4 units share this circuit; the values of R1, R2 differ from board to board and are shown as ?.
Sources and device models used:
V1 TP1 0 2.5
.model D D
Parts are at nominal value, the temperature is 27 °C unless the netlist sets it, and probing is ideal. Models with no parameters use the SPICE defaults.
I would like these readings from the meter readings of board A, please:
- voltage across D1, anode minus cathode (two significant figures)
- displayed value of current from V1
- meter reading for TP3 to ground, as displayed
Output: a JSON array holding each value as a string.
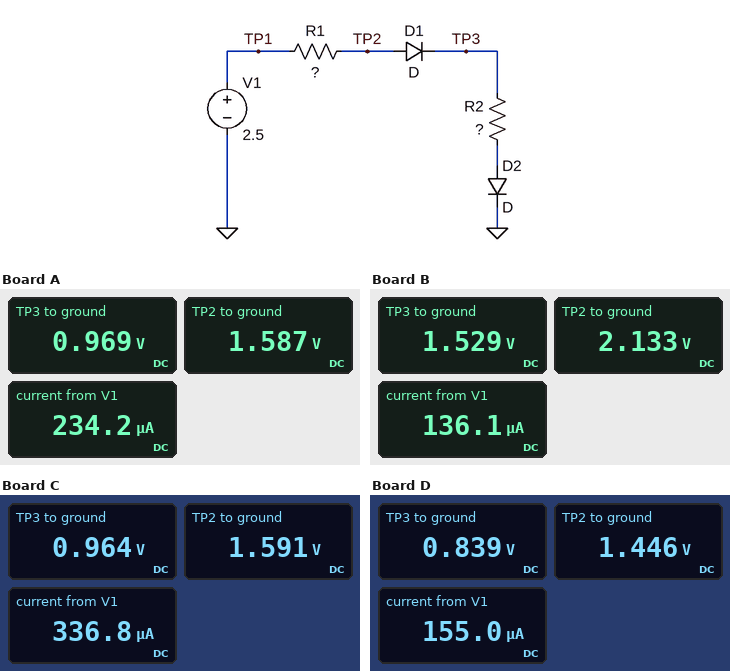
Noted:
["620 mV", "234.2 µA", "0.969 V"]
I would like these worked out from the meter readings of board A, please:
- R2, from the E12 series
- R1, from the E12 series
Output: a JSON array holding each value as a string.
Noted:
["1.5 kΩ", "3.9 kΩ"]
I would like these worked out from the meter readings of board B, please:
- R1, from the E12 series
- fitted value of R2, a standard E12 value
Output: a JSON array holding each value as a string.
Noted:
["2.7 kΩ", "6.8 kΩ"]
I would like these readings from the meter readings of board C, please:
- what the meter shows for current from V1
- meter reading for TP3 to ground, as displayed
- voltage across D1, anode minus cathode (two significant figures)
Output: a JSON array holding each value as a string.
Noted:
["336.8 µA", "0.964 V", "630 mV"]
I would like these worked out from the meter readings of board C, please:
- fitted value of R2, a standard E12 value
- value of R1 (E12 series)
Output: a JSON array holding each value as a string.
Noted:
["1 kΩ", "2.7 kΩ"]
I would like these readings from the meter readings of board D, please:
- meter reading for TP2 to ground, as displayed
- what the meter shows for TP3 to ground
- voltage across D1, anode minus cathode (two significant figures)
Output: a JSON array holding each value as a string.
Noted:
["1.446 V", "0.839 V", "610 mV"]
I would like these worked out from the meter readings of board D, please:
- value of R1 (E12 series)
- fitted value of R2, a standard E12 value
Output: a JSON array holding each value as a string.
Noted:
["6.8 kΩ", "1.5 kΩ"]
